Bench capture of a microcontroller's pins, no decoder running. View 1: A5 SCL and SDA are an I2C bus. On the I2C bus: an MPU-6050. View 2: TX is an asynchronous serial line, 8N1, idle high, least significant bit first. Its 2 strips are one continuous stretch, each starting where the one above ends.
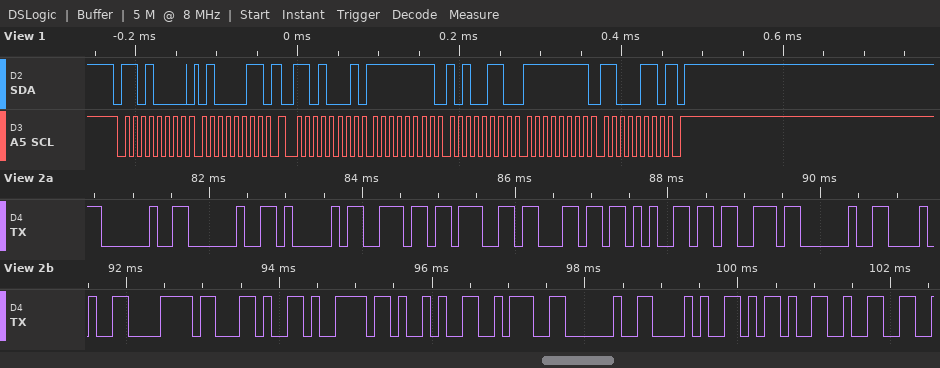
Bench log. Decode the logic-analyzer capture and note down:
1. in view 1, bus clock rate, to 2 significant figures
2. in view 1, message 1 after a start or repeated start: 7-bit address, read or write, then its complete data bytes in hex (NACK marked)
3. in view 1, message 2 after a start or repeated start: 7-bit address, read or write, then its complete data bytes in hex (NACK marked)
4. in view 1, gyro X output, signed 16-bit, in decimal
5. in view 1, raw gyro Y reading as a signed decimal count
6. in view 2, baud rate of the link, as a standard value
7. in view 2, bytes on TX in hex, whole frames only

100 kHz
0x68 write: 43
0x68 read: FF A6 FF C6 NACK
-90
-58
9600 baud
20 20 41 6E 67 6C 65 73 20 28 78 2C 79 29 3A 20 28 2D 32
